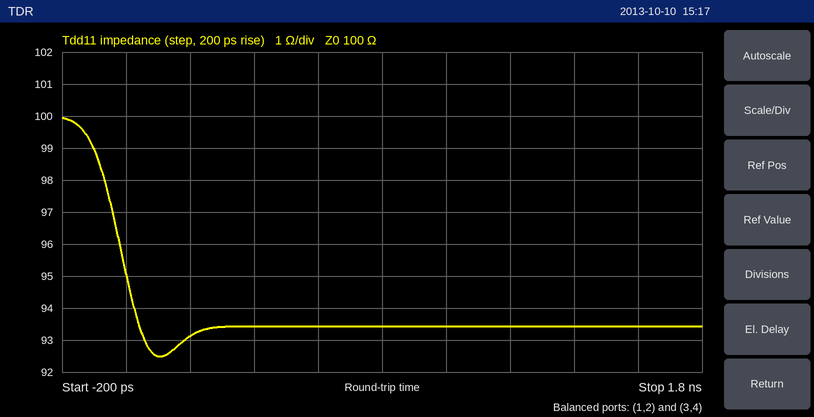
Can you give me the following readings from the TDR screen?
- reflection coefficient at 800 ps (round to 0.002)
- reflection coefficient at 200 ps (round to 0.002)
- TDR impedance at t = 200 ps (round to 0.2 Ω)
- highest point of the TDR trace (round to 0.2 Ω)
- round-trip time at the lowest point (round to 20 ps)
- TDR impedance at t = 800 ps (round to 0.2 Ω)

-0.034
-0.036
93.2 Ω
100.0 Ω
100 ps
93.4 Ω
